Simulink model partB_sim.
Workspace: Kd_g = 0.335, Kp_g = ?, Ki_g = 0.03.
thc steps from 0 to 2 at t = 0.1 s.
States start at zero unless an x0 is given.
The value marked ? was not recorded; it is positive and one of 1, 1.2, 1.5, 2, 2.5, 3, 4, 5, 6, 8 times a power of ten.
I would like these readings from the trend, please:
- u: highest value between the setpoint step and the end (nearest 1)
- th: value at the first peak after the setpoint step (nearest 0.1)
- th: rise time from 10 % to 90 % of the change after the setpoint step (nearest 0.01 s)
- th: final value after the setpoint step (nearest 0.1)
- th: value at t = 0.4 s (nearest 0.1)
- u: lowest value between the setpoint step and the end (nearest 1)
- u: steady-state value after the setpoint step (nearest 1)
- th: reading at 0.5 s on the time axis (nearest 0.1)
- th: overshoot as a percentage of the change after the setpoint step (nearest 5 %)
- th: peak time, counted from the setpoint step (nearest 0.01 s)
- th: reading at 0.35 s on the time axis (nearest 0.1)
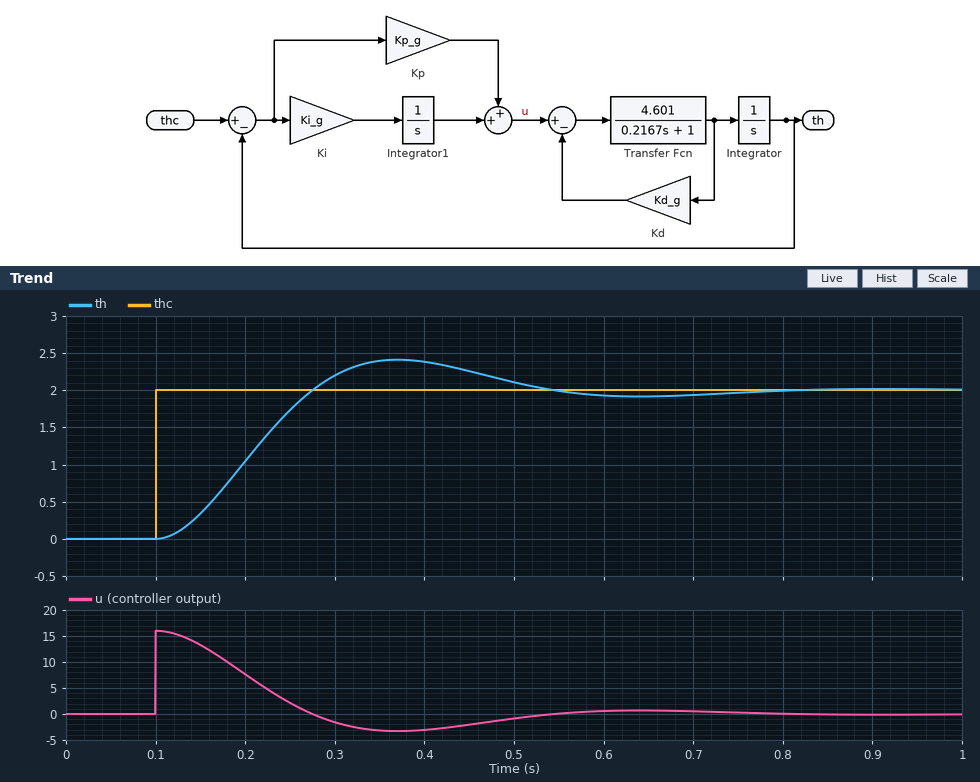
16
2.4
0.12 s
2.0
2.4
-3
0
2.1
20 %
0.27 s
2.4
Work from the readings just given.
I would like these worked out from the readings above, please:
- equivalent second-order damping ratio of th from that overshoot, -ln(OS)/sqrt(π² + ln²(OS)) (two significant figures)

0.46
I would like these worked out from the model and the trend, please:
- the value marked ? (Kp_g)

8
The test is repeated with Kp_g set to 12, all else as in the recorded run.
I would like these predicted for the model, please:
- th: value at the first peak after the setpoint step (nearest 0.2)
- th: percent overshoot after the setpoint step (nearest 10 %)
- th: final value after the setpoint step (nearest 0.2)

2.6
30 %
2.0
